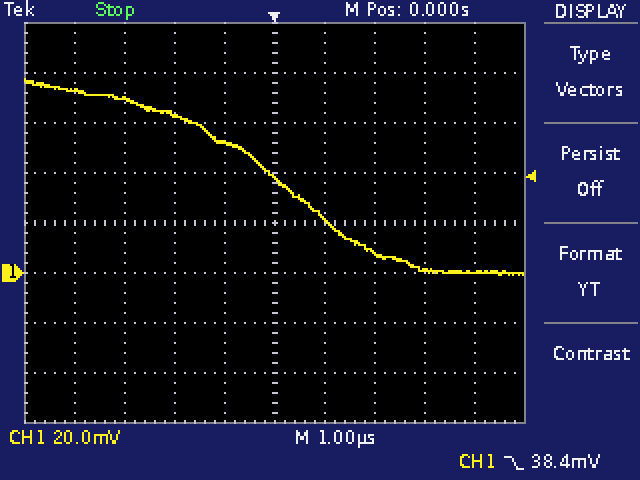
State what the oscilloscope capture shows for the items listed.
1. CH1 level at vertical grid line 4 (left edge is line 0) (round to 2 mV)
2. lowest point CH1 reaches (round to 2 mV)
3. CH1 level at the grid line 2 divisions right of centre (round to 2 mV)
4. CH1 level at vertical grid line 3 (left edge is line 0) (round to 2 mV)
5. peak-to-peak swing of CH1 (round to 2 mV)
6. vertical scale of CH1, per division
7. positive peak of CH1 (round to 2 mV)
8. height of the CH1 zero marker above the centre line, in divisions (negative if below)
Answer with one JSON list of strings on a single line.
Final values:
["52 mV", "0 mV", "8 mV", "64 mV", "78 mV", "20 mV", "78 mV", "-1.0 div"]
